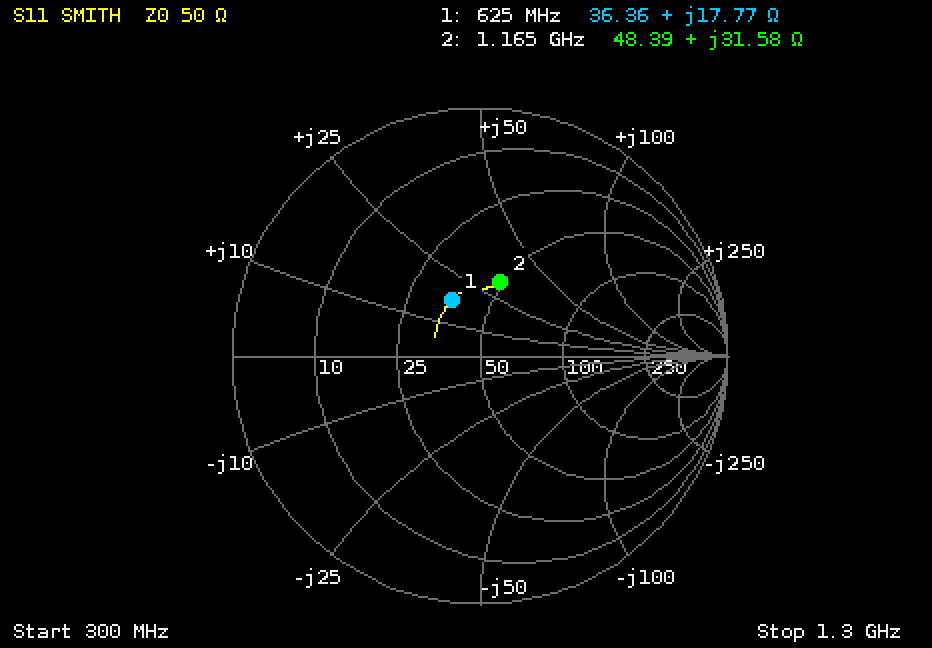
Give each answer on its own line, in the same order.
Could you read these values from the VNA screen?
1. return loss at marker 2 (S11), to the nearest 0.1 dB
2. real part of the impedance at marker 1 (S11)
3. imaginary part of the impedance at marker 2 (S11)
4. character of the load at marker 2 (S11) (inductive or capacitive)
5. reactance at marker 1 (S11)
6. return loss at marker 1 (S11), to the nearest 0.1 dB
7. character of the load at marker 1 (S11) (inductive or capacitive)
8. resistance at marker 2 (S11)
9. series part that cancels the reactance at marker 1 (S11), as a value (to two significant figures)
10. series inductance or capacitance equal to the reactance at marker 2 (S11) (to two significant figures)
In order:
10.3 dB
36.36 Ω
+31.58 Ω
inductive
+17.77 Ω
11.9 dB
inductive
48.39 Ω
14 pF
4.3 nH
